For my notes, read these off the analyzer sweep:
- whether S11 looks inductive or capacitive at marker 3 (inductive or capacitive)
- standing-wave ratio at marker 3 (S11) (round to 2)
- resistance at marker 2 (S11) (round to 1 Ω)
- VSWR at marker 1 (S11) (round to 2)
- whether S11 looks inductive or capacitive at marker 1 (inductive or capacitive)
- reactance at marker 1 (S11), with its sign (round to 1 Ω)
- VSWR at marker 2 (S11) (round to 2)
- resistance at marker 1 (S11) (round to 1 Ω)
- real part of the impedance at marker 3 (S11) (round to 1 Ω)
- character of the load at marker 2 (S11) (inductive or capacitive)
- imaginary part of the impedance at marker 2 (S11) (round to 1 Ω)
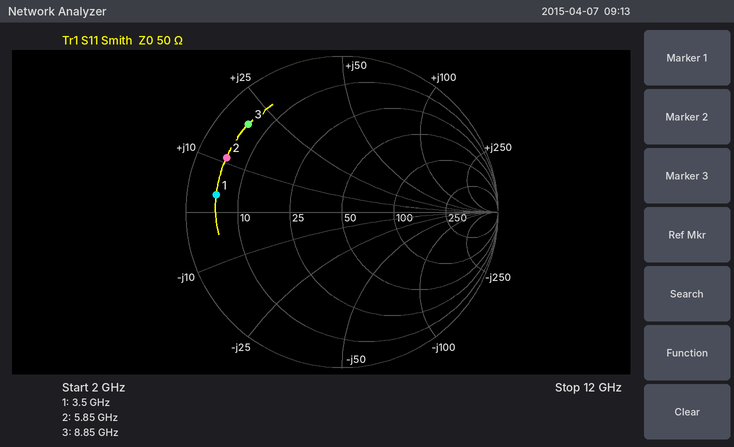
inductive
10
5 Ω
10
inductive
+3 Ω
10
5 Ω
6 Ω
inductive
+11 Ω
